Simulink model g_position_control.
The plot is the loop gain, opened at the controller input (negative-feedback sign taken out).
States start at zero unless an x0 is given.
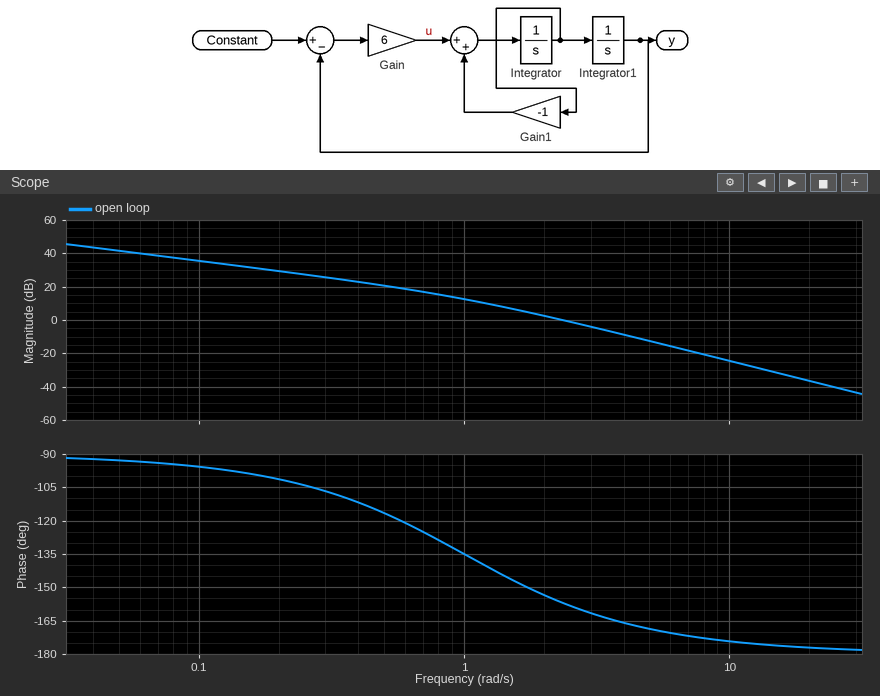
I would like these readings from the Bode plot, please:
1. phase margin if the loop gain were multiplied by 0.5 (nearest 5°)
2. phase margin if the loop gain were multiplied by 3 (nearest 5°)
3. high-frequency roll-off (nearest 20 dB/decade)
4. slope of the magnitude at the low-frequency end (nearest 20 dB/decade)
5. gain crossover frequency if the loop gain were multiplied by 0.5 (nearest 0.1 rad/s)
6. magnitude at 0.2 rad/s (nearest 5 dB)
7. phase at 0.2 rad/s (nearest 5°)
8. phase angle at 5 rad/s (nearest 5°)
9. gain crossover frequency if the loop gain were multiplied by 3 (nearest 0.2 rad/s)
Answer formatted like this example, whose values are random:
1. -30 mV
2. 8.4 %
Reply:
1. 30°
2. 15°
3. -40 dB/decade
4. -20 dB/decade
5. 1.6 rad/s
6. 30 dB
7. -100°
8. -170°
9. 4.2 rad/s
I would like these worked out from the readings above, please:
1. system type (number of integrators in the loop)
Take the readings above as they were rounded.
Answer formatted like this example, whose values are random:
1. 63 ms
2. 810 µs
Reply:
1. 1
